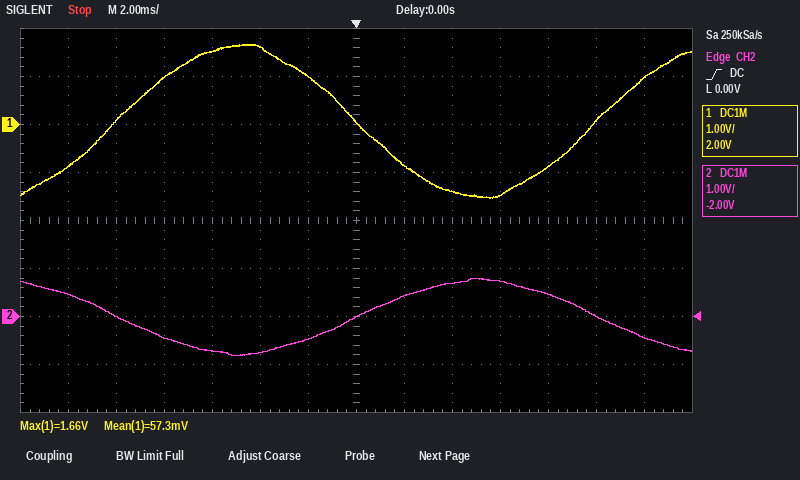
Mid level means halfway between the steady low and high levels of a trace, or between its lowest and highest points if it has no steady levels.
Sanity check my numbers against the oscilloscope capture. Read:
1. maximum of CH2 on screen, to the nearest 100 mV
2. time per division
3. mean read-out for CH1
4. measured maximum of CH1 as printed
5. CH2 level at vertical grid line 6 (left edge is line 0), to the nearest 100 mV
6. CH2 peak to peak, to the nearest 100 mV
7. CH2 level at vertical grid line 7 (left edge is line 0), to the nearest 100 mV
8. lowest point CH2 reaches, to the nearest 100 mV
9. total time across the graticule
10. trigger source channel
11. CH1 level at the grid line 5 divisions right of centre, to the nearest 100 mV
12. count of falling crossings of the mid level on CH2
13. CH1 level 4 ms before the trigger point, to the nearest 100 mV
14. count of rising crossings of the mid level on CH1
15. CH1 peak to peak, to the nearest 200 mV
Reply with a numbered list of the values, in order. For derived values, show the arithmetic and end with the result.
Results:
1. 800 mV
2. 2 ms
3. 57.3 mV
4. 1.66 V
5. -500 mV
6. 800 mV − (-800 mV) = 1.6 V
7. 0.0 V
8. -800 mV
9. 28 ms
10. CH2
11. 100 mV
12. 2
13. 1.6 V
14. 2
15. 3.2 V
